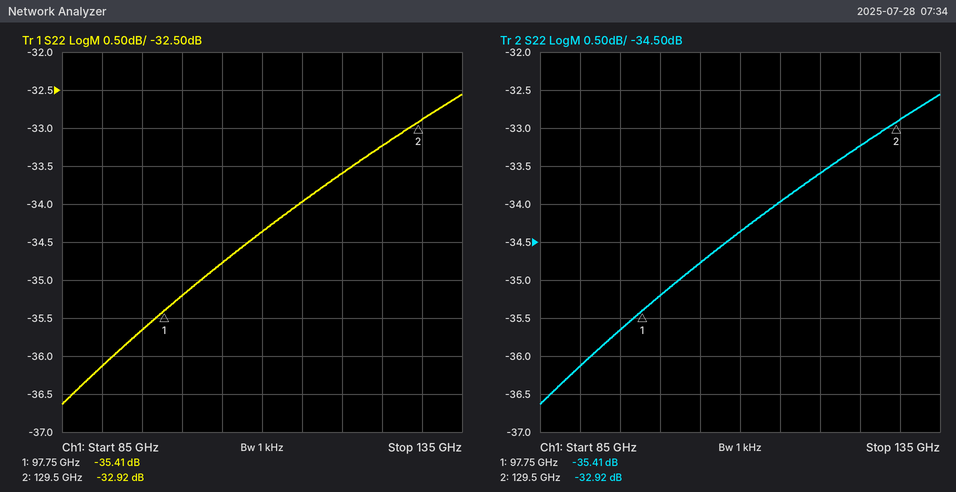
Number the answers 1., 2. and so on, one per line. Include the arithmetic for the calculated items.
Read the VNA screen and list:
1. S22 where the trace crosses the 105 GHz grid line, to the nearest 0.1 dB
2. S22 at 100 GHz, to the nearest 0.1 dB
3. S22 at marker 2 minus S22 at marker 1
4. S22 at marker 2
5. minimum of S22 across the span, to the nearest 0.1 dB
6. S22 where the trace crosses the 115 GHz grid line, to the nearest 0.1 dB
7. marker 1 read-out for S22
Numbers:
1. -34.8 dB
2. -35.2 dB
3. -32.92 − (-35.41) = 2.49 dB
4. -32.92 dB
5. -36.6 dB
6. -34.0 dB
7. -35.41 dB
